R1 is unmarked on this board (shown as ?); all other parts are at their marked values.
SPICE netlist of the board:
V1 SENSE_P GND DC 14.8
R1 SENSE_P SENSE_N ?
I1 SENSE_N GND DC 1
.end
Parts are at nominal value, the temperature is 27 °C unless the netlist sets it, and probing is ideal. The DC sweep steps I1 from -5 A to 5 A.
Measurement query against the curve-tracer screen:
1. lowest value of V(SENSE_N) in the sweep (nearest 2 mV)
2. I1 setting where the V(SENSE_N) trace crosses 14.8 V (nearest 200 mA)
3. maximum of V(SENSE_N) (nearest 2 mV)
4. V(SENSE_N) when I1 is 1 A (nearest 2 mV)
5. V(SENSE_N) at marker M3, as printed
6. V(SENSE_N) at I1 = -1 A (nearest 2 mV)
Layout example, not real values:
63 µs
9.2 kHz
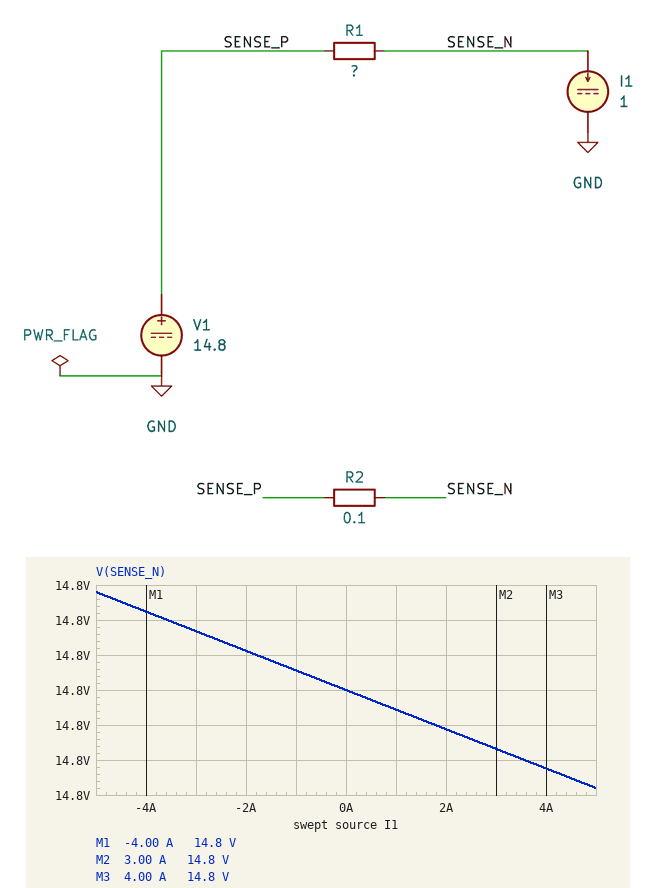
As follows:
14.772 V
0 A
14.828 V
14.794 V
14.8 V
14.806 V
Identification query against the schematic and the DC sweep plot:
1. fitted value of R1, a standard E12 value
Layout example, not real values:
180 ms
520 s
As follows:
5.6 mΩ
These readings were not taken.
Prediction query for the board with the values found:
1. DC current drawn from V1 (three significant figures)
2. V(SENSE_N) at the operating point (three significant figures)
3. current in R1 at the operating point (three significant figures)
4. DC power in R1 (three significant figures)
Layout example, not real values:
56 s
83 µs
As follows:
1.00 A
14.8 V
1.00 A
5.60 mW
